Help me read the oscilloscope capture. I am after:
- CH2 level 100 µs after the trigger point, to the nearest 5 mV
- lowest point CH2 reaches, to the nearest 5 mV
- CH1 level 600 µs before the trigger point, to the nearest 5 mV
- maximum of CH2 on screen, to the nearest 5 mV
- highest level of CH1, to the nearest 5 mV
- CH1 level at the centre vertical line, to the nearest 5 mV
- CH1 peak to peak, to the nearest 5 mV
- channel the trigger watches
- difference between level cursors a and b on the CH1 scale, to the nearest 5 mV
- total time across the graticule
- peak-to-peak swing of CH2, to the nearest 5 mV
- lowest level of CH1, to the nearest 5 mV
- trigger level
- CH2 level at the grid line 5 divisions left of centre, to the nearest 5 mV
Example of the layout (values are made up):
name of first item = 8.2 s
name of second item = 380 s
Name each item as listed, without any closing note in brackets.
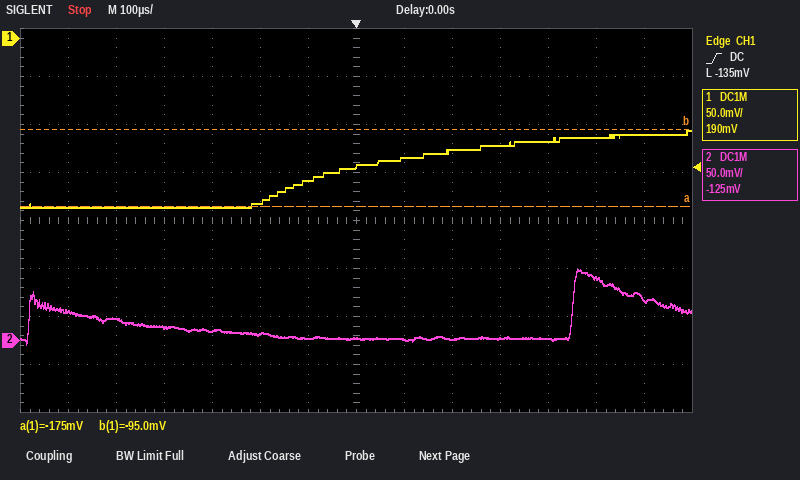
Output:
CH2 level 100 µs after the trigger point, to the nearest 5 mV = 0 mV
lowest point CH2 reaches, to the nearest 5 mV = -5 mV
CH1 level 600 µs before the trigger point, to the nearest 5 mV = -175 mV
maximum of CH2 on screen, to the nearest 5 mV = 75 mV
highest level of CH1, to the nearest 5 mV = -95 mV
CH1 level at the centre vertical line, to the nearest 5 mV = -135 mV
CH1 peak to peak, to the nearest 5 mV = 80 mV
channel the trigger watches = CH1
difference between level cursors a and b on the CH1 scale, to the nearest 5 mV = 80 mV
total time across the graticule = 1.4 ms
peak-to-peak swing of CH2, to the nearest 5 mV = 80 mV
lowest level of CH1, to the nearest 5 mV = -175 mV
trigger level = -135 mV
CH2 level at the grid line 5 divisions left of centre, to the nearest 5 mV = 20 mV
